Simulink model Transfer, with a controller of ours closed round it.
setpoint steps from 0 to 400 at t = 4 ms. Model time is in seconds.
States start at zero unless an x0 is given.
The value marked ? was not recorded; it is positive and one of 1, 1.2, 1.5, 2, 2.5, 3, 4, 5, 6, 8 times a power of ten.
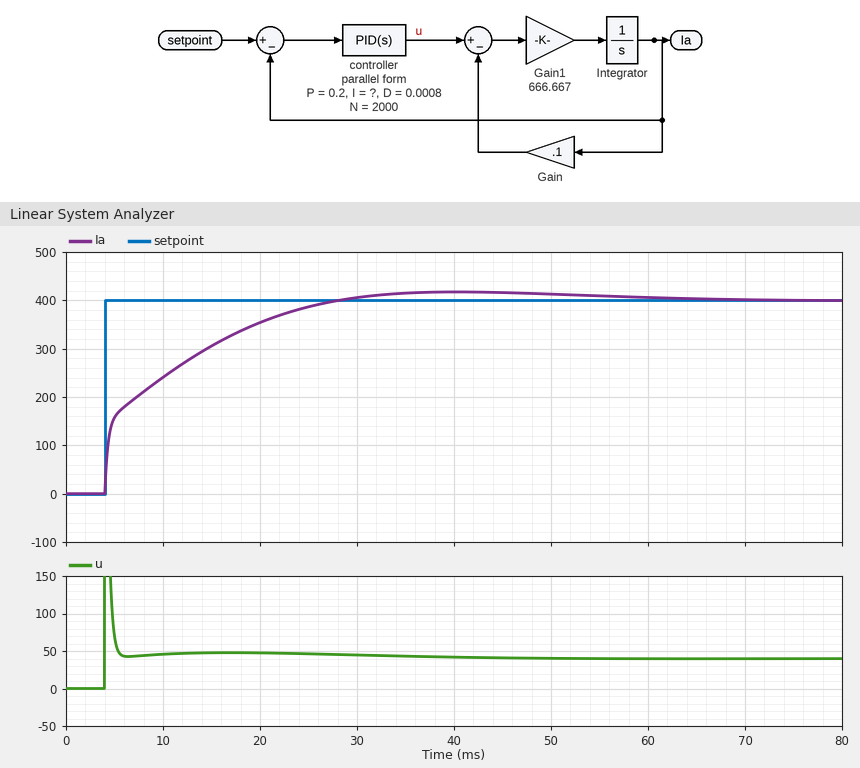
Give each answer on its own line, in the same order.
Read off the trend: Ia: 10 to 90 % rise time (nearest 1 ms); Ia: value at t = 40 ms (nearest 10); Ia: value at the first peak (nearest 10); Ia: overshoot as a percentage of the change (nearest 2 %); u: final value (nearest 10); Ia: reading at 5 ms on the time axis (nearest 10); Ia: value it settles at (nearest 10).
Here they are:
17 ms
420
420
4 %
40
160
400
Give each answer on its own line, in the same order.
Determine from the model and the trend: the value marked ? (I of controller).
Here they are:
20
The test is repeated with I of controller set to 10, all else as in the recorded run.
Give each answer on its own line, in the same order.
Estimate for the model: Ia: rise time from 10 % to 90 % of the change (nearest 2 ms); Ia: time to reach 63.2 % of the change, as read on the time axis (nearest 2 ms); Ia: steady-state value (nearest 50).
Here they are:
28 ms
12 ms
400
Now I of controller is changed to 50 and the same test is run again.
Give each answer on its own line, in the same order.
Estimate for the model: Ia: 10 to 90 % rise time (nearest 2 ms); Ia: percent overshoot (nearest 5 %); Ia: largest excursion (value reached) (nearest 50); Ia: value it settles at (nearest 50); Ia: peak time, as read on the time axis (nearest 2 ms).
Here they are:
10 ms
15 %
450
400
24 ms
